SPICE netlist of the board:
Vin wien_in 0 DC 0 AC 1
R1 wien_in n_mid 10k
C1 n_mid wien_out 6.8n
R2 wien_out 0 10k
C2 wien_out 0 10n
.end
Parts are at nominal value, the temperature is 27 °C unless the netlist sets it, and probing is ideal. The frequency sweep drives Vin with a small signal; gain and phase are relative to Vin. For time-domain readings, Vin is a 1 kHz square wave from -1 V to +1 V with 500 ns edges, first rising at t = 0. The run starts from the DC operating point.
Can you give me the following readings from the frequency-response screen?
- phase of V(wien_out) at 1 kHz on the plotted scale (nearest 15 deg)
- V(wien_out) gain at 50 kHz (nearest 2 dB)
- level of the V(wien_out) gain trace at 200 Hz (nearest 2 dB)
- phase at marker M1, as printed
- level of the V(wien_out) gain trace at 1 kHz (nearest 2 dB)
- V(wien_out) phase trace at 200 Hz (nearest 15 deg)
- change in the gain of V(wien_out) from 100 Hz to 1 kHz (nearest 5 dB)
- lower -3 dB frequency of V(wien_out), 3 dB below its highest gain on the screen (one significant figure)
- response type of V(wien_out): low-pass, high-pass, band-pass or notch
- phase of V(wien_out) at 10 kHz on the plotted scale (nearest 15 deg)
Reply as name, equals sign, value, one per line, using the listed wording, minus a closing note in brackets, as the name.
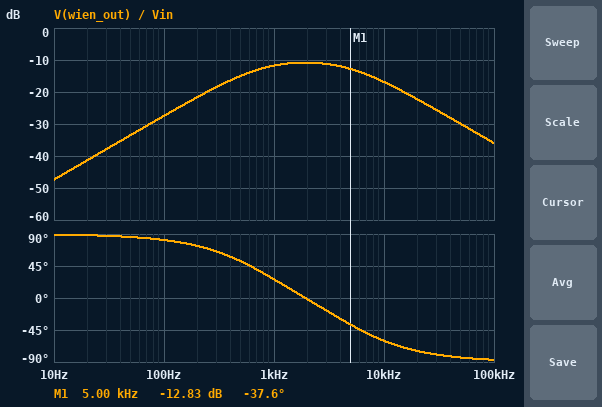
phase of V(wien_out) at 1 kHz on the plotted scale = 30 deg
V(wien_out) gain at 50 kHz = -30 dB
level of the V(wien_out) gain trace at 200 Hz = -22 dB
phase at marker M1, as printed = -37.6 deg
level of the V(wien_out) gain trace at 1 kHz = -12 dB
V(wien_out) phase trace at 200 Hz = 75 deg
change in the gain of V(wien_out) from 100 Hz to 1 kHz = 15 dB
lower -3 dB frequency of V(wien_out), 3 dB below its highest gain on the screen = 600 Hz
response type of V(wien_out): low-pass, high-pass, band-pass or notch = band-pass
phase of V(wien_out) at 10 kHz on the plotted scale = -60 deg
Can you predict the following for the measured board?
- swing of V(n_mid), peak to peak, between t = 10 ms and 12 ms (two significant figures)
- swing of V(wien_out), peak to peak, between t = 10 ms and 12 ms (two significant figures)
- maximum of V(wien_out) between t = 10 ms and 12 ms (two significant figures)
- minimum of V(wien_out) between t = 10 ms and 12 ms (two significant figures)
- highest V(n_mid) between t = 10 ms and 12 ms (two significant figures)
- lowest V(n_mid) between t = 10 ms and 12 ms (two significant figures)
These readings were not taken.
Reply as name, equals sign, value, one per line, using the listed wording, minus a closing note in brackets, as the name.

swing of V(n_mid), peak to peak, between t = 10 ms and 12 ms = 1.9 V
swing of V(wien_out), peak to peak, between t = 10 ms and 12 ms = 850 mV
maximum of V(wien_out) between t = 10 ms and 12 ms = 430 mV
minimum of V(wien_out) between t = 10 ms and 12 ms = -430 mV
highest V(n_mid) between t = 10 ms and 12 ms = 970 mV
lowest V(n_mid) between t = 10 ms and 12 ms = -970 mV
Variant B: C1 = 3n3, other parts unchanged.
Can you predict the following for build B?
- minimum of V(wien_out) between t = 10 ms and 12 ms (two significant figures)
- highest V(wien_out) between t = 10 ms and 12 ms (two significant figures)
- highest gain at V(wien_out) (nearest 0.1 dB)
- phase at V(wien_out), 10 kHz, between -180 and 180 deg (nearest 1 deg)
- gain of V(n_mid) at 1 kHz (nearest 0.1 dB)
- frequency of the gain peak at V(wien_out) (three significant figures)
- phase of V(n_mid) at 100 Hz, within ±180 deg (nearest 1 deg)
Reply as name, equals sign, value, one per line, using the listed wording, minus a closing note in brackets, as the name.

minimum of V(wien_out) between t = 10 ms and 12 ms = -310 mV
highest V(wien_out) between t = 10 ms and 12 ms = 310 mV
highest gain at V(wien_out) = -14.0 dB
phase at V(wien_out), 10 kHz, between -180 and 180 deg = -49 deg
gain of V(n_mid) at 1 kHz = -0.4 dB
frequency of the gain peak at V(wien_out) = 2.77 kHz
phase of V(n_mid) at 100 Hz, within ±180 deg = -1 deg
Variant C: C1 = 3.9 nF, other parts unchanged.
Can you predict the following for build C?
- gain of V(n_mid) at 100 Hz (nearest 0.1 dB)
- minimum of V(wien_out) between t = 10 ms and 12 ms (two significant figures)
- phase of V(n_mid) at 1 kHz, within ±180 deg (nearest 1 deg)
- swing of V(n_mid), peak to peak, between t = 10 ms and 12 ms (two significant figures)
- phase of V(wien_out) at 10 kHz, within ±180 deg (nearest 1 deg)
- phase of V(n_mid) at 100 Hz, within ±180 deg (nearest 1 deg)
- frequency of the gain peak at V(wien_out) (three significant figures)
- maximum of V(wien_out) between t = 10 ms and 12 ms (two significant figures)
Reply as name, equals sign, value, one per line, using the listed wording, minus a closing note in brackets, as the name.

gain of V(n_mid) at 100 Hz = 0 dB
minimum of V(wien_out) between t = 10 ms and 12 ms = -340 mV
phase of V(n_mid) at 1 kHz, within ±180 deg = -12 deg
swing of V(n_mid), peak to peak, between t = 10 ms and 12 ms = 2.0 V
phase of V(wien_out) at 10 kHz, within ±180 deg = -52 deg
phase of V(n_mid) at 100 Hz, within ±180 deg = -1 deg
frequency of the gain peak at V(wien_out) = 2.55 kHz
maximum of V(wien_out) between t = 10 ms and 12 ms = 340 mV
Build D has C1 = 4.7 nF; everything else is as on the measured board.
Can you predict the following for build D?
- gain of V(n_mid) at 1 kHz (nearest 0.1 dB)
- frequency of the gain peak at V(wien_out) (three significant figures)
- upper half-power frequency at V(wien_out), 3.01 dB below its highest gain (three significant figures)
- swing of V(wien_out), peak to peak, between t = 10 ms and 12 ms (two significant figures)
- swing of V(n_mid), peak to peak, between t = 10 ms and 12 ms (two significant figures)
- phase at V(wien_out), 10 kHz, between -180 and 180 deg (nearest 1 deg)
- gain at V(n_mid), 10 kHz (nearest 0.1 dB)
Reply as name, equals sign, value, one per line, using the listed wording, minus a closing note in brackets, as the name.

gain of V(n_mid) at 1 kHz = -0.6 dB
frequency of the gain peak at V(wien_out) = 2.32 kHz
upper half-power frequency at V(wien_out), 3.01 dB below its highest gain = 7.31 kHz
swing of V(wien_out), peak to peak, between t = 10 ms and 12 ms = 740 mV
swing of V(n_mid), peak to peak, between t = 10 ms and 12 ms = 2.0 V
phase at V(wien_out), 10 kHz, between -180 and 180 deg = -55 deg
gain at V(n_mid), 10 kHz = -7.2 dB
